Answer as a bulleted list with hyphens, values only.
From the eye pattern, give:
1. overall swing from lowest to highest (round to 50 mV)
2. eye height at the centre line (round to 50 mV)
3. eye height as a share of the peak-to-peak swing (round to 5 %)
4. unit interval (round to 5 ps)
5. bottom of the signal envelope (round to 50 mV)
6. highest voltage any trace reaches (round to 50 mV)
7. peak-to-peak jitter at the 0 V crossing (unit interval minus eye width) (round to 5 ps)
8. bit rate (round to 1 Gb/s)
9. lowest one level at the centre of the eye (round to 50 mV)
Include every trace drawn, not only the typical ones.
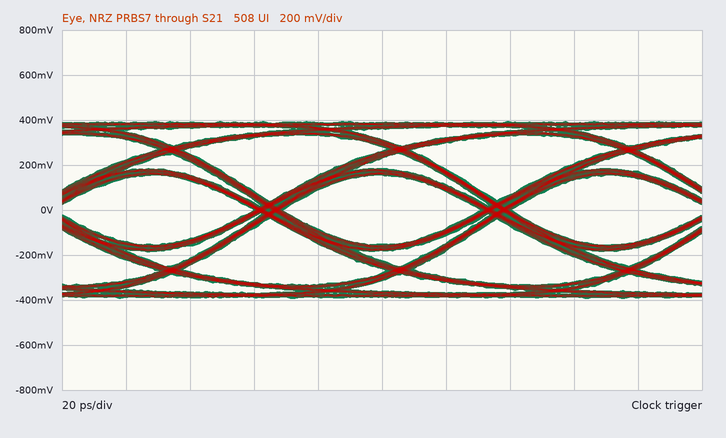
- 800 mV
- 300 mV
- 40 %
- 70 ps
- -400 mV
- 400 mV
- 10 ps
- 14 Gb/s
- 150 mV
